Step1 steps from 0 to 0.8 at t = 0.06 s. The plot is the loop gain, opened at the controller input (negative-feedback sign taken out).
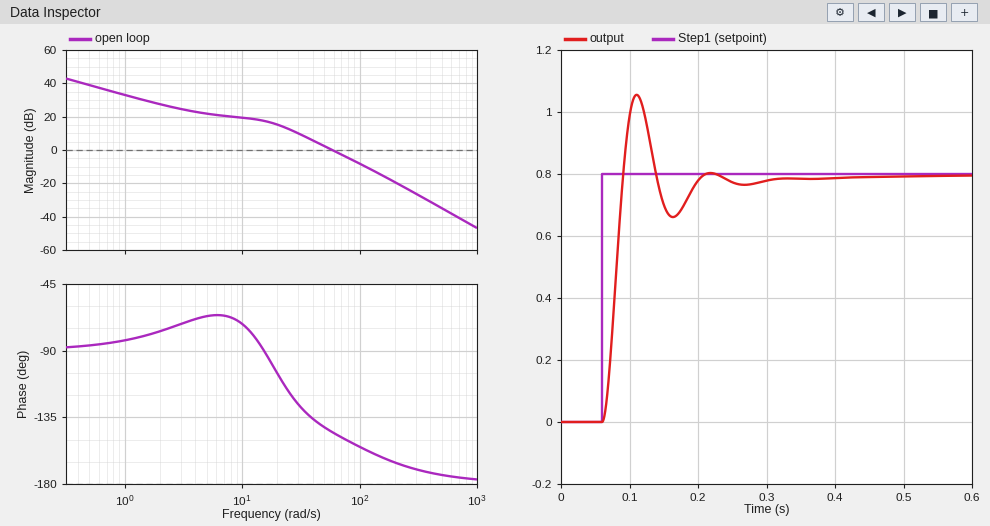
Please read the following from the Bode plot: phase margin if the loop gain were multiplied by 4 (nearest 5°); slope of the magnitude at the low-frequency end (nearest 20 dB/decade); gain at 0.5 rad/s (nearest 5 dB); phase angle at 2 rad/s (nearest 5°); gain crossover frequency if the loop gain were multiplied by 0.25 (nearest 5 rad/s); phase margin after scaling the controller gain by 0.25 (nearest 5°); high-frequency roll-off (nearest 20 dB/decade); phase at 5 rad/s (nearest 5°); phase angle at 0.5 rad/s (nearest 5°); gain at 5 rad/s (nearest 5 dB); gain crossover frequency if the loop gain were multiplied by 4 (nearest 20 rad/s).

20°
-20 dB/decade
40 dB
-75°
25 rad/s
60°
-40 dB/decade
-65°
-85°
20 dB
120 rad/s
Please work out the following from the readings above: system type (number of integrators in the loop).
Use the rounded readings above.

1
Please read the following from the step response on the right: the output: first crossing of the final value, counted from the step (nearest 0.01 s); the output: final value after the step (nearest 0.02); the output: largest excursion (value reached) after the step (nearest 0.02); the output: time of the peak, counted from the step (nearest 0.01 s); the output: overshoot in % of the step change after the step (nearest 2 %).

0.03 s
0.80
1.06
0.05 s
32 %
